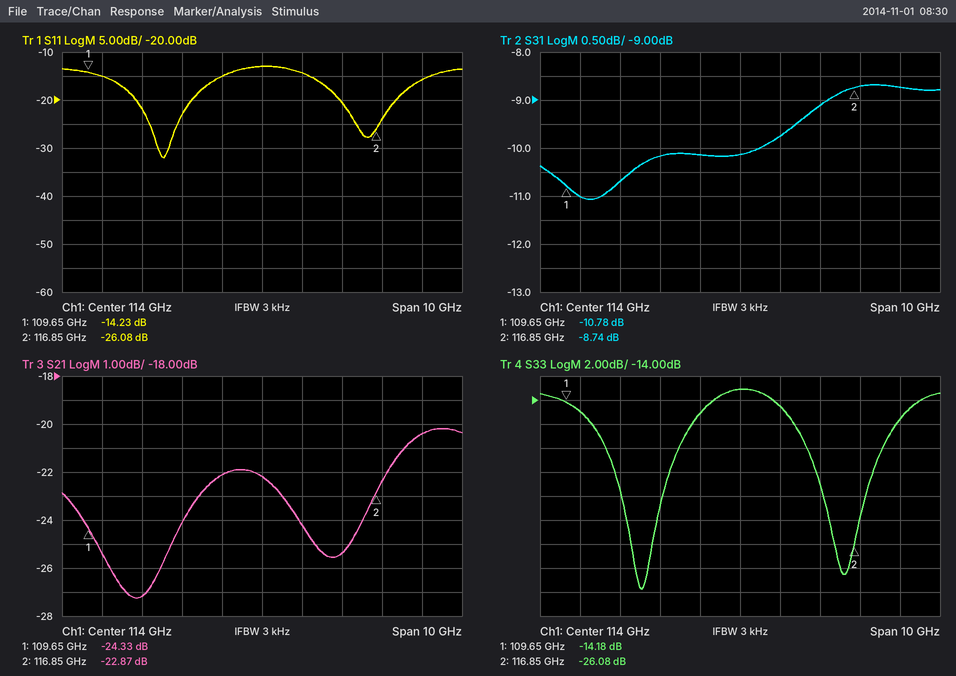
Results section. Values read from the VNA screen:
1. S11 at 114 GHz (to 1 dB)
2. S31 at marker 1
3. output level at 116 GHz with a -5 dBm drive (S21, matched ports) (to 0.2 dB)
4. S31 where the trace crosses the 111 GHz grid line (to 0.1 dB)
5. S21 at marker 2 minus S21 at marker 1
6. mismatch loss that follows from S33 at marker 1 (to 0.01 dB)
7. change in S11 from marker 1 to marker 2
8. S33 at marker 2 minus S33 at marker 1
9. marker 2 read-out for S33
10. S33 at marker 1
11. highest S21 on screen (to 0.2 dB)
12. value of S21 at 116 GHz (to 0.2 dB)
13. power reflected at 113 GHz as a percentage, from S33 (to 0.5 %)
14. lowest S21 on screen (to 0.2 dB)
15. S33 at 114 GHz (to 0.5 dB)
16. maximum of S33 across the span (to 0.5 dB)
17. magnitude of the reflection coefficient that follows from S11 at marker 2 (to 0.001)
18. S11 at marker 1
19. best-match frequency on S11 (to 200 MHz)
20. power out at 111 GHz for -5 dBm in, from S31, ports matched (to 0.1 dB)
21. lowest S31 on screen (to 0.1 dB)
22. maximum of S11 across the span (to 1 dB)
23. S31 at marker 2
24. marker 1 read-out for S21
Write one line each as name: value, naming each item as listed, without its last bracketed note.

S11 at 114 GHz: -13 dB
S31 at marker 1: -10.78 dB
output level at 116 GHz with a -5 dBm drive (S21, matched ports): -30.4 dBm
S31 where the trace crosses the 111 GHz grid line: -10.7 dB
S21 at marker 2 minus S21 at marker 1: 1.46 dB
mismatch loss that follows from S33 at marker 1: 0.17 dB
change in S11 from marker 1 to marker 2: -11.85 dB
S33 at marker 2 minus S33 at marker 1: -11.90 dB
marker 2 read-out for S33: -26.08 dB
S33 at marker 1: -14.18 dB
highest S21 on screen: -20.2 dB
value of S21 at 116 GHz: -25.4 dB
power reflected at 113 GHz as a percentage, from S33: 3.0 %
lowest S21 on screen: -27.2 dB
S33 at 114 GHz: -13.0 dB
maximum of S33 across the span: -13.0 dB
magnitude of the reflection coefficient that follows from S11 at marker 2: 0.050
S11 at marker 1: -14.23 dB
best-match frequency on S11: 111.6 GHz
power out at 111 GHz for -5 dBm in, from S31, ports matched: -15.7 dBm
lowest S31 on screen: -11.1 dB
maximum of S11 across the span: -13 dB
S31 at marker 2: -8.74 dB
marker 1 read-out for S21: -24.33 dB
